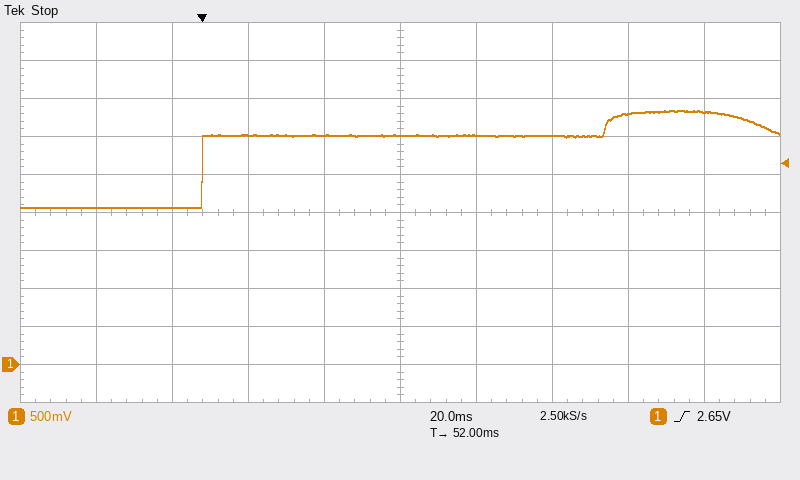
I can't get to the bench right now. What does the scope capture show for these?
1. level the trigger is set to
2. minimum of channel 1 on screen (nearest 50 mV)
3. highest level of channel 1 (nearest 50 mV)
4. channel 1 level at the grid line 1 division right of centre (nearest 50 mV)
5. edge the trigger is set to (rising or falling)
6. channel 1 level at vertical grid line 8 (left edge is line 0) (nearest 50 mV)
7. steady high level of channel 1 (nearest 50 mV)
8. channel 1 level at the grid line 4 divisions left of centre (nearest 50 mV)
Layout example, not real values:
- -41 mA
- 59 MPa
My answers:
- 2.65 V
- 2.05 V
- 3.35 V
- 3.00 V
- rising
- 3.30 V
- 3.00 V
- 2.05 V
